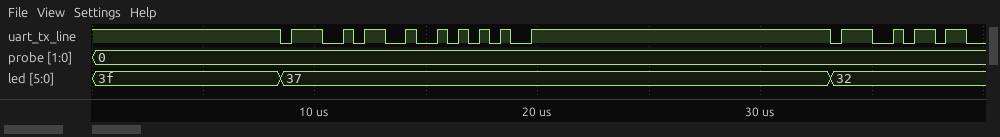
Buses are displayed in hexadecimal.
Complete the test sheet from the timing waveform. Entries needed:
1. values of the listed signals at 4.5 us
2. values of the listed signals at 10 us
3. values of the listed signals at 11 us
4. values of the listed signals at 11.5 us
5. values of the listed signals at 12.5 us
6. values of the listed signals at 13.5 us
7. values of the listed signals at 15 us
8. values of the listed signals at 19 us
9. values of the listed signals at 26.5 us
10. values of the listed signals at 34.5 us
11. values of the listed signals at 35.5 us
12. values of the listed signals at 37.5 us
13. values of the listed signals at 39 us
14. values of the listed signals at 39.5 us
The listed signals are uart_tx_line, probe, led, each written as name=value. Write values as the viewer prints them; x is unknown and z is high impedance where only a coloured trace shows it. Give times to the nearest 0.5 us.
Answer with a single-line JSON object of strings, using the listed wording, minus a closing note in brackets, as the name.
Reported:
{"values of the listed signals at 4.5 us": "uart_tx_line=1, probe=0, led=3f", "values of the listed signals at 10 us": "uart_tx_line=1, probe=0, led=37", "values of the listed signals at 11 us": "uart_tx_line=0, probe=0, led=37", "values of the listed signals at 11.5 us": "uart_tx_line=1, probe=0, led=37", "values of the listed signals at 12.5 us": "uart_tx_line=1, probe=0, led=37", "values of the listed signals at 13.5 us": "uart_tx_line=0, probe=0, led=37", "values of the listed signals at 15 us": "uart_tx_line=0, probe=0, led=37", "values of the listed signals at 19 us": "uart_tx_line=0, probe=0, led=37", "values of the listed signals at 26.5 us": "uart_tx_line=1, probe=0, led=37", "values of the listed signals at 34.5 us": "uart_tx_line=1, probe=0, led=32", "values of the listed signals at 35.5 us": "uart_tx_line=0, probe=0, led=32", "values of the listed signals at 37.5 us": "uart_tx_line=1, probe=0, led=32", "values of the listed signals at 39 us": "uart_tx_line=1, probe=0, led=32", "values of the listed signals at 39.5 us": "uart_tx_line=0, probe=0, led=32"}
